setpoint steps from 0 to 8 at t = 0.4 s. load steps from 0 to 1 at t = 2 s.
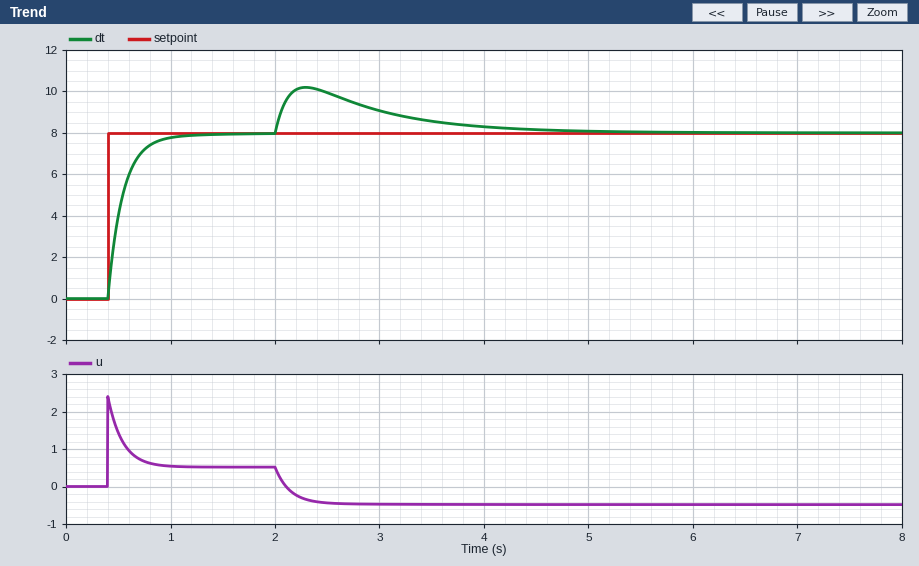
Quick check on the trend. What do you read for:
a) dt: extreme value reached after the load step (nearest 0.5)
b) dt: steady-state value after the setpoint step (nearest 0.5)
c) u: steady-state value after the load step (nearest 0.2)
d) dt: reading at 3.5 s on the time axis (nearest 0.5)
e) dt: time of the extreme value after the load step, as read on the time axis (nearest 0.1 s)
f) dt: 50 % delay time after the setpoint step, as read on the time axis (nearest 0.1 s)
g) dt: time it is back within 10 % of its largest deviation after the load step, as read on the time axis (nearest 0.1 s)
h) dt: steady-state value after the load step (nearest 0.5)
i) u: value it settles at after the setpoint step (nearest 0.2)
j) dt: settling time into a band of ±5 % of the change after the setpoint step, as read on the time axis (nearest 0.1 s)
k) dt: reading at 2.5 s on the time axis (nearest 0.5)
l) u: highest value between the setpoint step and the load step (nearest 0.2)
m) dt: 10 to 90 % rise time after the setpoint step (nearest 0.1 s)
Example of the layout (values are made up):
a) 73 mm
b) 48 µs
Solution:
a) 10.0
b) 8.0
c) -0.4
d) 8.5
e) 2.3 s
f) 0.5 s
g) 4.2 s
h) 8.0
i) 0.6
j) 0.9 s
k) 10.0
l) 2.4
m) 0.3 s
